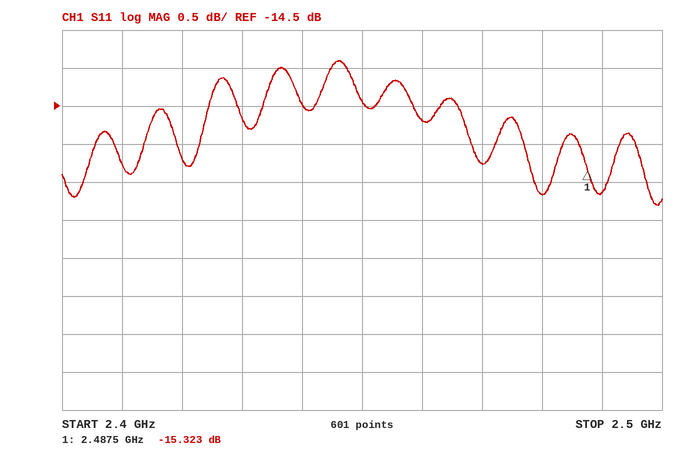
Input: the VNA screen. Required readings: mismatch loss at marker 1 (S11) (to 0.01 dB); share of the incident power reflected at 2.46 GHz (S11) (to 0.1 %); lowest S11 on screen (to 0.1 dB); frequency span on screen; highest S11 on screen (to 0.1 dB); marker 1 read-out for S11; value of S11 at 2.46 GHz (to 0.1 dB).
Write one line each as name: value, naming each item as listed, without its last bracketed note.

mismatch loss at marker 1 (S11): 0.13 dB
share of the incident power reflected at 2.46 GHz (S11): 3.4 %
lowest S11 on screen: -15.8 dB
frequency span on screen: 100 MHz
highest S11 on screen: -13.9 dB
marker 1 read-out for S11: -15.323 dB
value of S11 at 2.46 GHz: -14.7 dB
